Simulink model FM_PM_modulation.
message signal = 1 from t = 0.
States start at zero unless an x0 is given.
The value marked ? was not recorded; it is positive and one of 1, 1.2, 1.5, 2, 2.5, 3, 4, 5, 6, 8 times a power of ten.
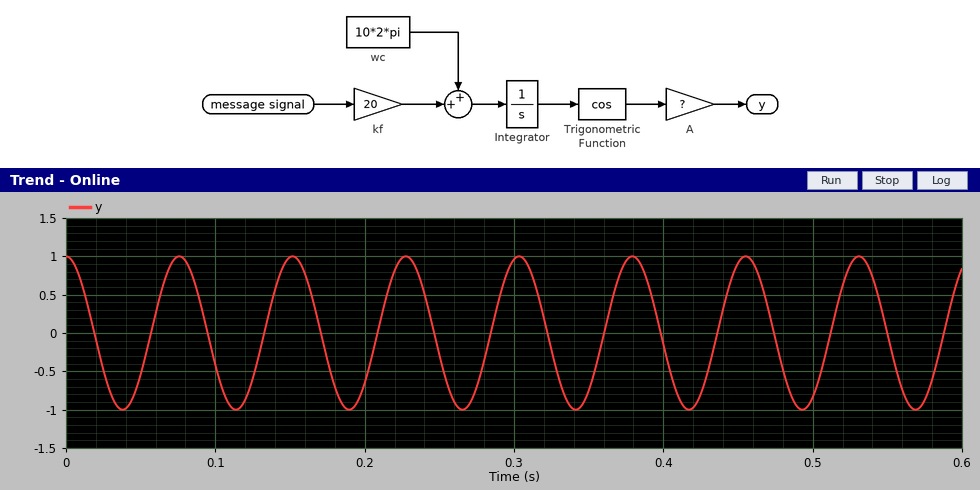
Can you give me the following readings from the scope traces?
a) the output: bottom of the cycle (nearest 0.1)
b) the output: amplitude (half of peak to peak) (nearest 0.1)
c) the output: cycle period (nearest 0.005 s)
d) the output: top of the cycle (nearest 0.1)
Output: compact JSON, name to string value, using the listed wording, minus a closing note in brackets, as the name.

{"the output: bottom of the cycle": "-1.0", "the output: amplitude (half of peak to peak)": "1.0", "the output: cycle period": "0.075 s", "the output: top of the cycle": "1.0"}
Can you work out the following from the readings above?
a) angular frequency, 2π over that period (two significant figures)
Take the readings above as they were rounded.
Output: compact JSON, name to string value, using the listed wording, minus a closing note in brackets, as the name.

{"angular frequency, 2π over that period": "84 rad/s"}
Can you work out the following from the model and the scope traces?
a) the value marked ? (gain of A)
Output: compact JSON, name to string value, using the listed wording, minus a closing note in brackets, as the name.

{"the value marked ?": "1"}
